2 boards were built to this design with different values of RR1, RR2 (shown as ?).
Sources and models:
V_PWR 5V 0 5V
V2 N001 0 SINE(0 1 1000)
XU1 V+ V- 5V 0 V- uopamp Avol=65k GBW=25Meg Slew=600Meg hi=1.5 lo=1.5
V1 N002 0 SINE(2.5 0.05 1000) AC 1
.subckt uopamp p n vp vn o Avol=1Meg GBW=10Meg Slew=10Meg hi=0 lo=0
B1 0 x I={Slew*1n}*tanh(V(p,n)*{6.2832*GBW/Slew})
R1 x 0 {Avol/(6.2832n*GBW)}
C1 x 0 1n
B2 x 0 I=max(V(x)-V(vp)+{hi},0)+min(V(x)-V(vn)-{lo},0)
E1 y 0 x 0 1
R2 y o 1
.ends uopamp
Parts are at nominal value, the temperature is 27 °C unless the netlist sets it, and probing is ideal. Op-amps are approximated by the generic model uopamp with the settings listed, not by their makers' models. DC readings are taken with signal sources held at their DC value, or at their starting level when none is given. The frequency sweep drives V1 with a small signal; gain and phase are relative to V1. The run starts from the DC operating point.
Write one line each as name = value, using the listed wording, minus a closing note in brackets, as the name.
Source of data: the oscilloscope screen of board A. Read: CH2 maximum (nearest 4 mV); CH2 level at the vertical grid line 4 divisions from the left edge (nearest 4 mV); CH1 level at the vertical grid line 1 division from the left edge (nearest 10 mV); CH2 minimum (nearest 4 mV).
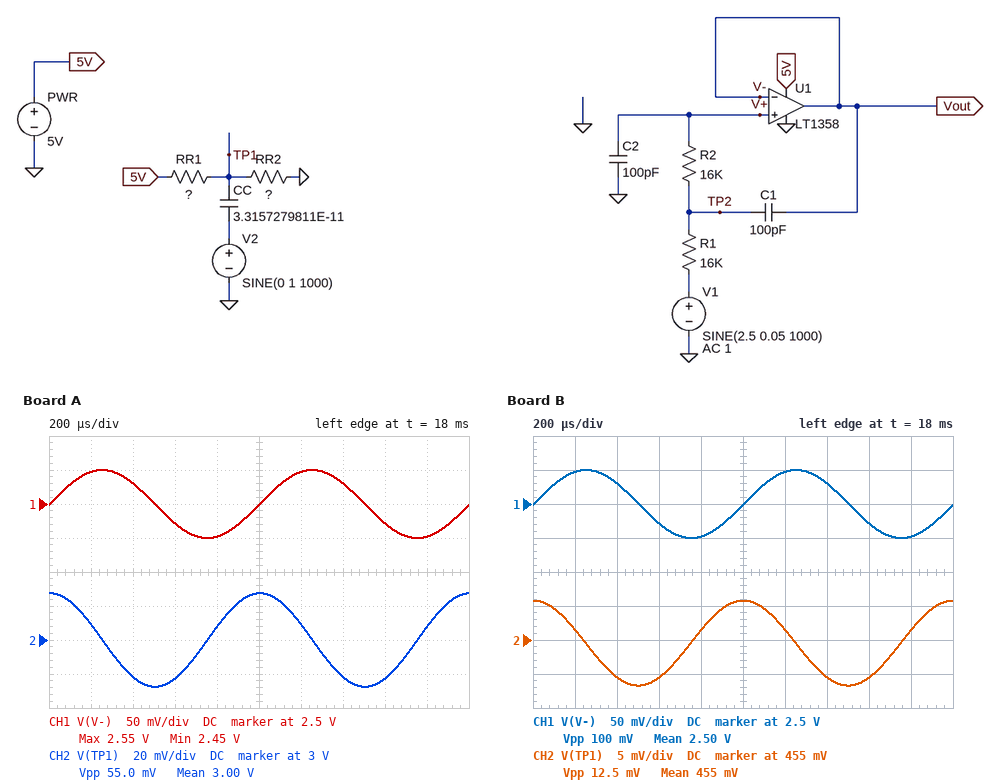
CH2 maximum = 3.028 V
CH2 level at the vertical grid line 4 divisions from the left edge = 3.008 V
CH1 level at the vertical grid line 1 division from the left edge = 2.55 V
CH2 minimum = 2.972 V
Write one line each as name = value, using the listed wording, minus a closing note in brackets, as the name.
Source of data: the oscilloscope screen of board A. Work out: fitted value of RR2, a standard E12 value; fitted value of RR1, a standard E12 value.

fitted value of RR2, a standard E12 value = 330 kΩ
fitted value of RR1, a standard E12 value = 220 kΩ
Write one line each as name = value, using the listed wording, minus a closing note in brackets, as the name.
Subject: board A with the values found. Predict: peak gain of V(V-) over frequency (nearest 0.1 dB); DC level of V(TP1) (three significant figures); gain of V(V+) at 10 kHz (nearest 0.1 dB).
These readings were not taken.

peak gain of V(V-) over frequency = 0 dB
DC level of V(TP1) = 3.00 V
gain of V(V+) at 10 kHz = -0.1 dB
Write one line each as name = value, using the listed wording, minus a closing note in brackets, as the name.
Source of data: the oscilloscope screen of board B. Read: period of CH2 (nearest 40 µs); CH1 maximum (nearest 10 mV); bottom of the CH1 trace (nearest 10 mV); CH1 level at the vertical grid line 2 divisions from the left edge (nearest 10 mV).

period of CH2 = 1.00 ms
CH1 maximum = 2.55 V
bottom of the CH1 trace = 2.45 V
CH1 level at the vertical grid line 2 divisions from the left edge = 2.53 V
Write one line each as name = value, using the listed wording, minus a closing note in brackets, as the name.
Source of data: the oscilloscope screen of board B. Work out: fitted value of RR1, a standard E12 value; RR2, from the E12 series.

fitted value of RR1, a standard E12 value = 330 kΩ
RR2, from the E12 series = 33 kΩ
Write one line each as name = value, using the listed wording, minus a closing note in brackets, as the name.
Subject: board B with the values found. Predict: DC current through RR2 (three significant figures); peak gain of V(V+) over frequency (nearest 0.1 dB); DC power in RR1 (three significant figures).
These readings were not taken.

DC current through RR2 = 13.8 µA
peak gain of V(V+) over frequency = 0 dB
DC power in RR1 = 62.6 µW
